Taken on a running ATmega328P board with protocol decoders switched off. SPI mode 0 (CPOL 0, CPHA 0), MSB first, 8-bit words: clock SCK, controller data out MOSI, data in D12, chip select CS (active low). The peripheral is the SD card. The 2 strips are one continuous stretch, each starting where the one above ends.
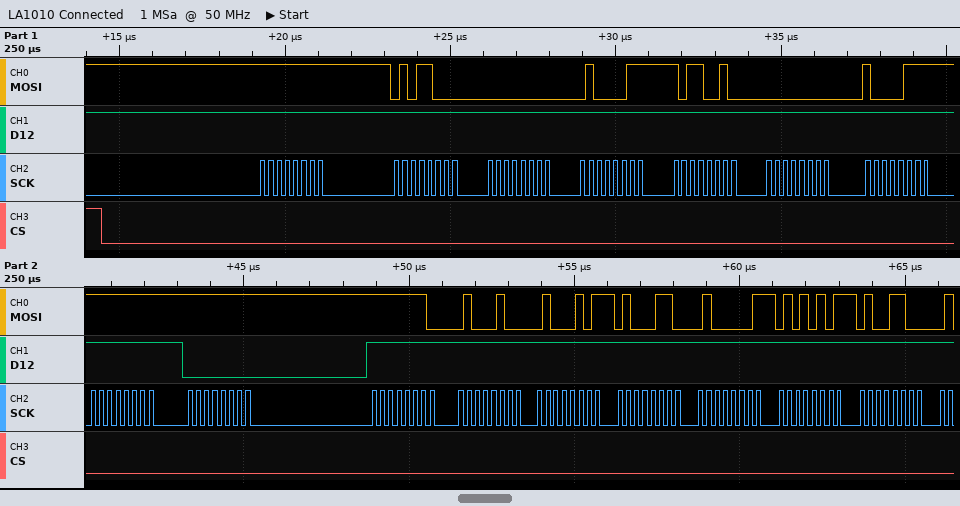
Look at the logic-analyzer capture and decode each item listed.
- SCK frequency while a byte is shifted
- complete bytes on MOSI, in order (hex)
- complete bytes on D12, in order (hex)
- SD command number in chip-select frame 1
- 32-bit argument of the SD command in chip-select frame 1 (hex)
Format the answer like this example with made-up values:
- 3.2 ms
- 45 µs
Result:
- 4 MHz
- 0xFF 0x58 0x00 0x43 0xB2 0x00 0x87 0xFF 0xFF 0xFE 0x44 0x45 0x46 0x41 0x55 0x4C
- 0xFF 0xFF 0xFF 0xFF 0xFF 0xFF 0xFF 0xFF 0x00 0xFF 0xFF 0xFF 0xFF 0xFF 0xFF 0xFF
- CMD24
- 0x0043B200
